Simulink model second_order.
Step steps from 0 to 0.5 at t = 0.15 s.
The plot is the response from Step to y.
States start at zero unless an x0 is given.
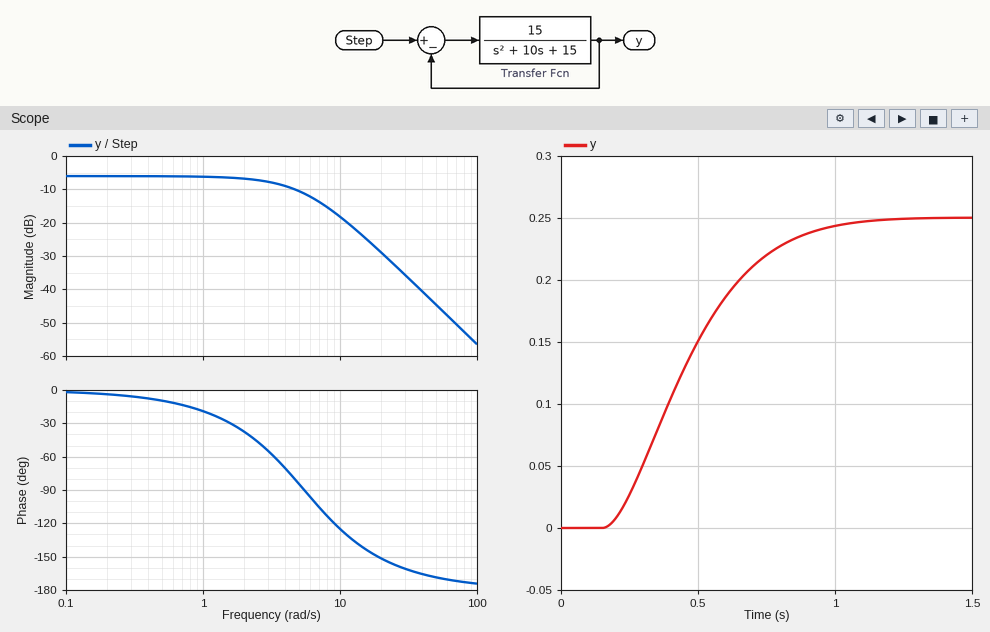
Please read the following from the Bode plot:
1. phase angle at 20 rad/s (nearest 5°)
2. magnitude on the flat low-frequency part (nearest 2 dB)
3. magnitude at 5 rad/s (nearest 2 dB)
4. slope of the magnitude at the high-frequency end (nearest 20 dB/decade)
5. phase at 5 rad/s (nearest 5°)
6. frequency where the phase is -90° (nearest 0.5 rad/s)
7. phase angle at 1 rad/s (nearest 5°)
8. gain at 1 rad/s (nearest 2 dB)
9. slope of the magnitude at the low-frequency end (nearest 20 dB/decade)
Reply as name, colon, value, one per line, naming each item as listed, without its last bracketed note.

phase angle at 20 rad/s: -150°
magnitude on the flat low-frequency part: -6 dB
magnitude at 5 rad/s: -10 dB
slope of the magnitude at the high-frequency end: -40 dB/decade
phase at 5 rad/s: -85°
frequency where the phase is -90°: 5.5 rad/s
phase angle at 1 rad/s: -20°
gain at 1 rad/s: -6 dB
slope of the magnitude at the low-frequency end: 0 dB/decade
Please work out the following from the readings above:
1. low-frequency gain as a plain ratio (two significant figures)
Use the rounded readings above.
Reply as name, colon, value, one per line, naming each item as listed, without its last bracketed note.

low-frequency gain as a plain ratio: 0.50
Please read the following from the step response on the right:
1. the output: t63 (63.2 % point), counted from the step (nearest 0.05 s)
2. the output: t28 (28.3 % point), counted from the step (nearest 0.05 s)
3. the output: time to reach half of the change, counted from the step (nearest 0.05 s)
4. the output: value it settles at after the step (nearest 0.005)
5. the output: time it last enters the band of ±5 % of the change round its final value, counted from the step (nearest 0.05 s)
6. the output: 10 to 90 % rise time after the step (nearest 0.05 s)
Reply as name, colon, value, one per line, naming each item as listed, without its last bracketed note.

the output: t63 (63.2 % point), counted from the step: 0.35 s
the output: t28 (28.3 % point), counted from the step: 0.20 s
the output: time to reach half of the change, counted from the step: 0.30 s
the output: value it settles at after the step: 0.250
the output: time it last enters the band of ±5 % of the change round its final value, counted from the step: 0.75 s
the output: 10 to 90 % rise time after the step: 0.55 s
